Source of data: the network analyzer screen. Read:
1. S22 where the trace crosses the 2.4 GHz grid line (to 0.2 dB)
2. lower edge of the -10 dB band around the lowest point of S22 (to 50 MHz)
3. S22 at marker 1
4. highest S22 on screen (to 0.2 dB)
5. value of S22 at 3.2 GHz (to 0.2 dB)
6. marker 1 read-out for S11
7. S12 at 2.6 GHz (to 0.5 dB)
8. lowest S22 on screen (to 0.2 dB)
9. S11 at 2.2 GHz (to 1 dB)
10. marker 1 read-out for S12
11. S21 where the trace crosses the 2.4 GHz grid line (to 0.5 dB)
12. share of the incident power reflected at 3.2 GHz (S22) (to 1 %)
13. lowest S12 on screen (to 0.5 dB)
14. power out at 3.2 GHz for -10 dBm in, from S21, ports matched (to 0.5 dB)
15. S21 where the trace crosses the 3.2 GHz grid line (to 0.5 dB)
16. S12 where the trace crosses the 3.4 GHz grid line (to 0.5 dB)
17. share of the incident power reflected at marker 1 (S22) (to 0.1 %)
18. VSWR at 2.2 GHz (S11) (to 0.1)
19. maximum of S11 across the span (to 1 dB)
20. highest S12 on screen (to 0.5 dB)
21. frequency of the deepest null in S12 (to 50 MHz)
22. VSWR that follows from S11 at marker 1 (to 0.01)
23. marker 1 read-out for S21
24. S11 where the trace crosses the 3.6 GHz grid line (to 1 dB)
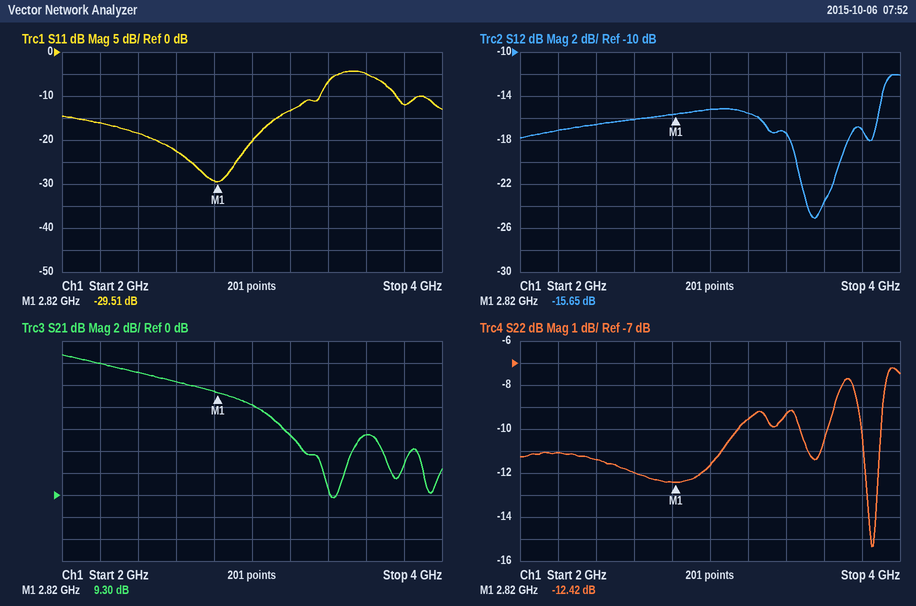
-11.4 dB
3.80 GHz
-12.42 dB
-7.2 dB
-9.6 dB
-29.51 dB
-16.0 dB
-15.4 dB
-16 dB
-15.65 dB
11.0 dB
11 %
-25.0 dB
-4.5 dBm
5.5 dB
-17.5 dB
5.7 %
1.4
-4 dB
-12.0 dB
3.55 GHz
1.07
9.30 dB
-5 dB
